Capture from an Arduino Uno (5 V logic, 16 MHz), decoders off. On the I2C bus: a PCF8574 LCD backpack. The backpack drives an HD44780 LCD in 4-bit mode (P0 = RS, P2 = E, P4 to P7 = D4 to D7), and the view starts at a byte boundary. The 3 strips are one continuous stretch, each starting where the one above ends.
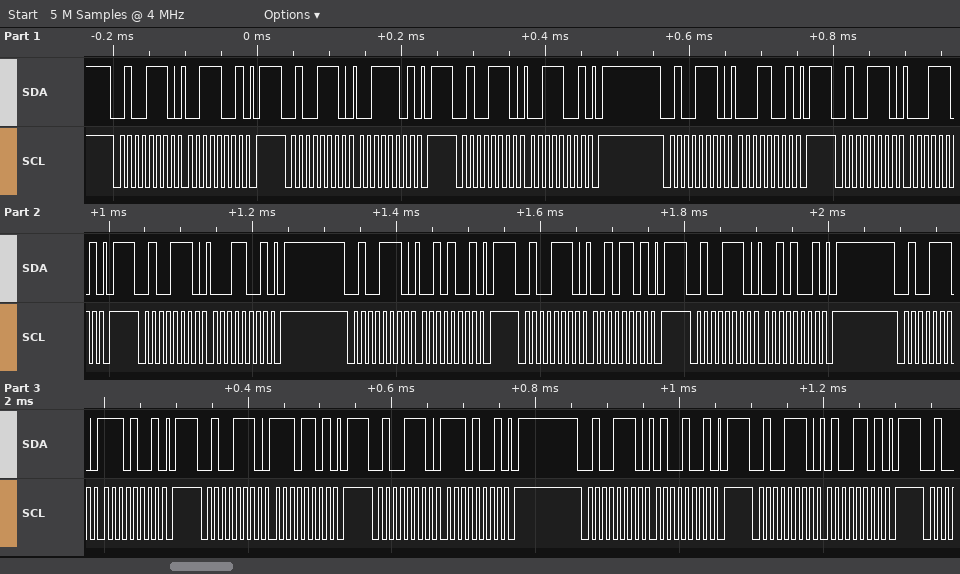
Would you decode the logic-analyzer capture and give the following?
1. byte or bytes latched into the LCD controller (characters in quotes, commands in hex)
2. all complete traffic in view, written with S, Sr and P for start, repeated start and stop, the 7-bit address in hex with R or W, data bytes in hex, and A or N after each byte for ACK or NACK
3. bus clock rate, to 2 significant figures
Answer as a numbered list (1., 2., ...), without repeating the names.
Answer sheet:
1. '1' '.'
2. S 27W A 39 A P S 27W A 3D A P S 27W A 39 A P S 27W A 19 A P S 27W A 1D A P S 27W A 19 A P S 27W A 29 A P S 27W A 2D A P S 27W A 29 A P S 27W A E9 A P S 27W A ED A P S 27W A E9 A P S 27W A 49 A P S 27W A 4D A P
3. 100 kHz
